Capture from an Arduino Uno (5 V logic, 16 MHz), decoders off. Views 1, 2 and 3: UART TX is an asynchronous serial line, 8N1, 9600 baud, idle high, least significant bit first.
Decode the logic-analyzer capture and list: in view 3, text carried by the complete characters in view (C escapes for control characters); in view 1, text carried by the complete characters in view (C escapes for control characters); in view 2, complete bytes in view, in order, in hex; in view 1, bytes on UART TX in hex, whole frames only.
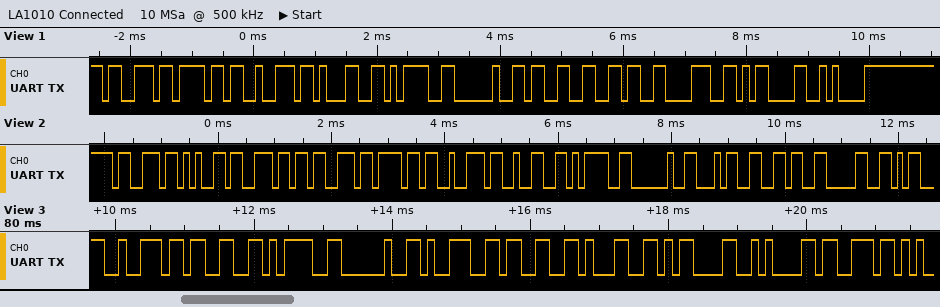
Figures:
"r3= 931\r\ns"
"sor1= 368\r\n"
73 65 6E 73 6F 72 32 3D 20 34 36 30
73 6F 72 31 3D 20 33 36 38 0D 0A
